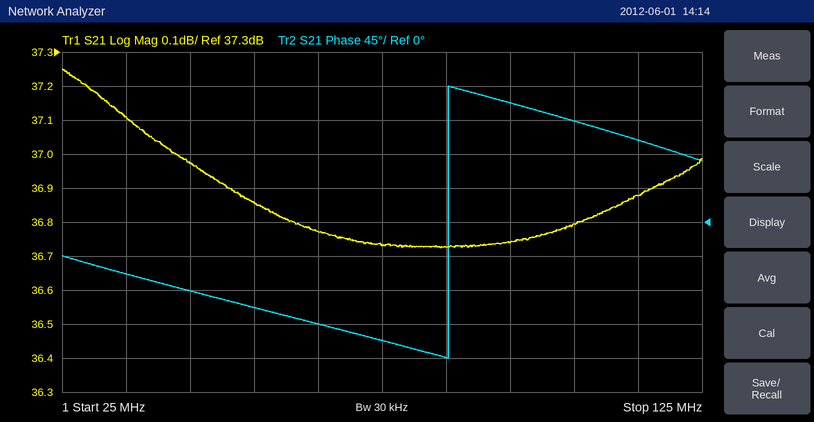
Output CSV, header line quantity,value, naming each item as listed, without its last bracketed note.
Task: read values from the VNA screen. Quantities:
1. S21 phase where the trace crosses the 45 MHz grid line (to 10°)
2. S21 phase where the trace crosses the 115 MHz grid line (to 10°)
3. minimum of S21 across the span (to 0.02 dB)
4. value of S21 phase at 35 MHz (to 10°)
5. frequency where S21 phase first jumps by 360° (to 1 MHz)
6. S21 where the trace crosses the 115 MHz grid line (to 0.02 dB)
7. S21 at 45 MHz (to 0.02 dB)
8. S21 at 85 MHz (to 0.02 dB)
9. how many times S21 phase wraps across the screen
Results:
quantity,value
S21 phase where the trace crosses the 45 MHz grid line,-90°
S21 phase where the trace crosses the 115 MHz grid line,110°
minimum of S21 across the span,36.72 dB
value of S21 phase at 35 MHz,-70°
frequency where S21 phase first jumps by 360°,85 MHz
S21 where the trace crosses the 115 MHz grid line,36.88 dB
S21 at 45 MHz,36.98 dB
S21 at 85 MHz,36.72 dB
how many times S21 phase wraps across the screen,1
